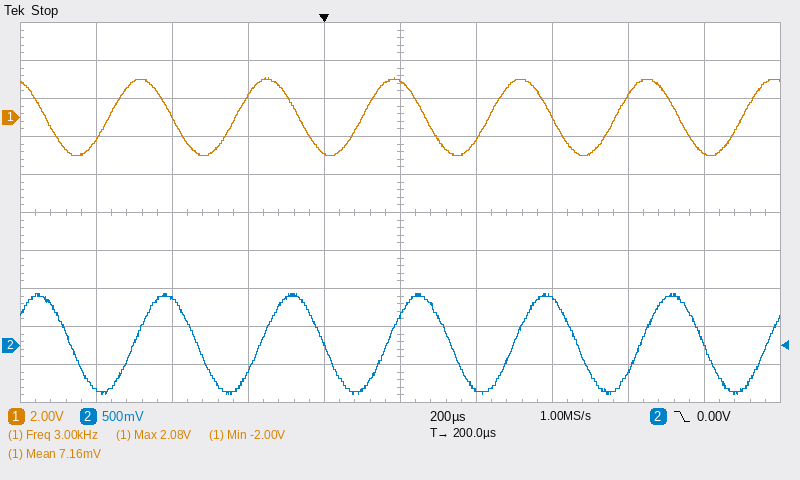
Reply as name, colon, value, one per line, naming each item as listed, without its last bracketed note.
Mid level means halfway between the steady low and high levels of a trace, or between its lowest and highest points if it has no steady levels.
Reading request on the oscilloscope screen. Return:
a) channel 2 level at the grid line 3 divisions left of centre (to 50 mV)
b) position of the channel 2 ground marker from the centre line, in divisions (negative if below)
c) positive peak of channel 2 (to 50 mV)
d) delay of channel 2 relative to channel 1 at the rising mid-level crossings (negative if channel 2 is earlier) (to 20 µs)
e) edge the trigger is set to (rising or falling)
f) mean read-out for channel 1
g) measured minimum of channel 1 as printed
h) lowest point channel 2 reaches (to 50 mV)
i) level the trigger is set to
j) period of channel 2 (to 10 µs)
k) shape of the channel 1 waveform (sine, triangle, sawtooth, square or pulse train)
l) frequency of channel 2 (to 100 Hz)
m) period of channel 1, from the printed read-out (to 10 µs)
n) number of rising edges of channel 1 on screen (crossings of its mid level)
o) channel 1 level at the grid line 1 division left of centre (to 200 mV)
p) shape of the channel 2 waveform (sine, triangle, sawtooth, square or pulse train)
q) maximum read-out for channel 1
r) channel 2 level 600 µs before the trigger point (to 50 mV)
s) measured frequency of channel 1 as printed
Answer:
channel 2 level at the grid line 3 divisions left of centre: 600 mV
position of the channel 2 ground marker from the centre line, in divisions: -3.5 div
positive peak of channel 2: 700 mV
delay of channel 2 relative to channel 1 at the rising mid-level crossings (negative if channel 2 is earlier): +60 µs
edge the trigger is set to: falling
mean read-out for channel 1: 7.16 mV
measured minimum of channel 1 as printed: -2.00 V
lowest point channel 2 reaches: -650 mV
level the trigger is set to: 0.00 V
period of channel 2: 330 µs
shape of the channel 1 waveform: sine
frequency of channel 2: 3.0 kHz
period of channel 1, from the printed read-out: 330 µs
number of rising edges of channel 1 on screen: 6
channel 1 level at the grid line 1 division left of centre: -1.8 V
shape of the channel 2 waveform: sine
maximum read-out for channel 1: 2.08 V
channel 2 level 600 µs before the trigger point: -550 mV
measured frequency of channel 1 as printed: 3.00 kHz
